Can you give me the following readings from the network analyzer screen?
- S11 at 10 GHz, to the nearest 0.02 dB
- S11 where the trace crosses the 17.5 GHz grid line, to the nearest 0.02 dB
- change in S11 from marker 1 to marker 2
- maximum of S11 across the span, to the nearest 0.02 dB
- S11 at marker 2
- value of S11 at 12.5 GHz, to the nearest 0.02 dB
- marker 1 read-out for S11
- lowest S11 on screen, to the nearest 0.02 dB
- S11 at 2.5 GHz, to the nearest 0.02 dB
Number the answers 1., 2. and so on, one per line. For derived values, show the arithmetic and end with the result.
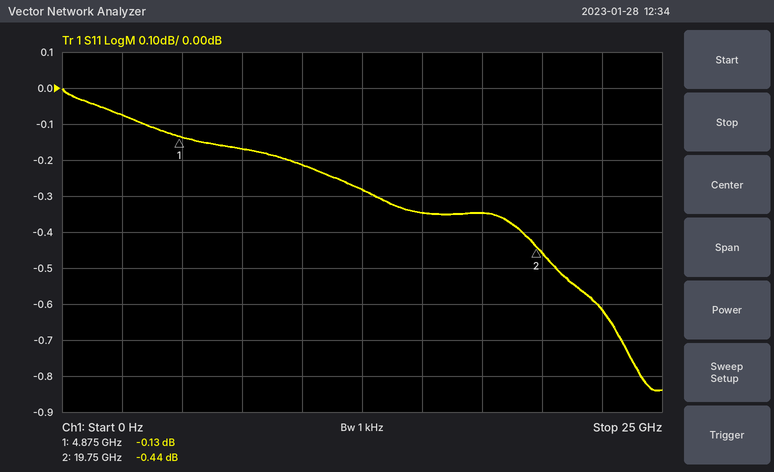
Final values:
1. -0.22 dB
2. -0.34 dB
3. -0.44 − (-0.13) = -0.31 dB
4. 0.00 dB
5. -0.44 dB
6. -0.28 dB
7. -0.13 dB
8. -0.84 dB
9. -0.08 dB
